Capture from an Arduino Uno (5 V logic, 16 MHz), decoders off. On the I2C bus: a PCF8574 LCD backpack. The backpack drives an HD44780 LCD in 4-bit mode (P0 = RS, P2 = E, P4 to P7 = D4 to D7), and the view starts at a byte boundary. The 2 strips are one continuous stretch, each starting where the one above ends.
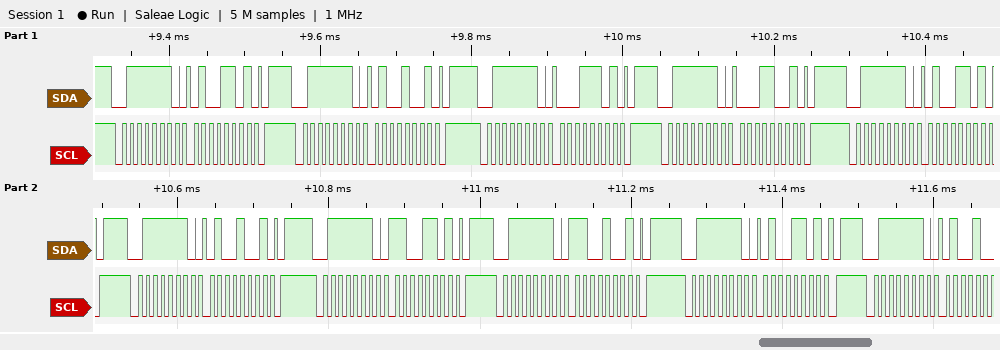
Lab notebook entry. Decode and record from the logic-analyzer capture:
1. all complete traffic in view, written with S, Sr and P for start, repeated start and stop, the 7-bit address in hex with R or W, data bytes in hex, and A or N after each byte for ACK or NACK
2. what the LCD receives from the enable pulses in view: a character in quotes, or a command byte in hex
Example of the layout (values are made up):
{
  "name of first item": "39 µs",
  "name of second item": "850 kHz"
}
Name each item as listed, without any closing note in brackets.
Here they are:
{
  "all complete traffic in view, written with S, Sr and P for start, repeated start and stop, the 7-bit address in hex with R or W, data bytes in hex, and A or N after each byte for ACK or NACK": "S 3FW A 4D A P S 3FW A 49 A P S 3FW A 1D A P S 3FW A 19 A P S 3FW A 4D A P S 3FW A 49 A P S 3FW A CD A P S 3FW A C9 A P S 3FW A 4D A P S 3FW A",
  "what the LCD receives from the enable pulses in view: a character in quotes, or a command byte in hex": "'A' 'L'"
}
